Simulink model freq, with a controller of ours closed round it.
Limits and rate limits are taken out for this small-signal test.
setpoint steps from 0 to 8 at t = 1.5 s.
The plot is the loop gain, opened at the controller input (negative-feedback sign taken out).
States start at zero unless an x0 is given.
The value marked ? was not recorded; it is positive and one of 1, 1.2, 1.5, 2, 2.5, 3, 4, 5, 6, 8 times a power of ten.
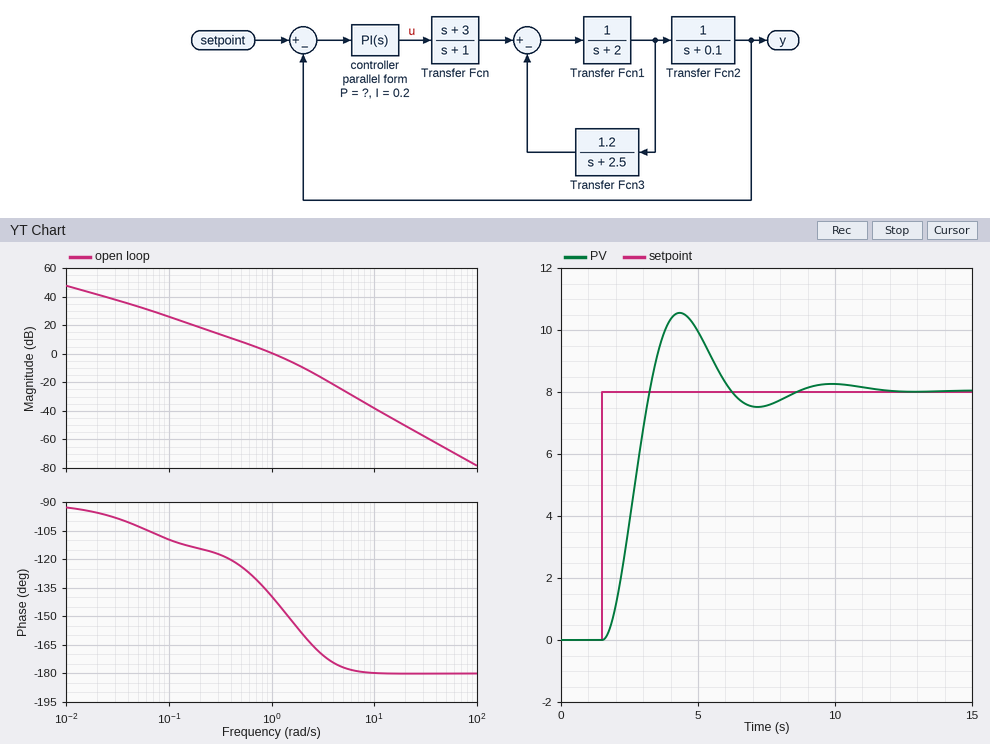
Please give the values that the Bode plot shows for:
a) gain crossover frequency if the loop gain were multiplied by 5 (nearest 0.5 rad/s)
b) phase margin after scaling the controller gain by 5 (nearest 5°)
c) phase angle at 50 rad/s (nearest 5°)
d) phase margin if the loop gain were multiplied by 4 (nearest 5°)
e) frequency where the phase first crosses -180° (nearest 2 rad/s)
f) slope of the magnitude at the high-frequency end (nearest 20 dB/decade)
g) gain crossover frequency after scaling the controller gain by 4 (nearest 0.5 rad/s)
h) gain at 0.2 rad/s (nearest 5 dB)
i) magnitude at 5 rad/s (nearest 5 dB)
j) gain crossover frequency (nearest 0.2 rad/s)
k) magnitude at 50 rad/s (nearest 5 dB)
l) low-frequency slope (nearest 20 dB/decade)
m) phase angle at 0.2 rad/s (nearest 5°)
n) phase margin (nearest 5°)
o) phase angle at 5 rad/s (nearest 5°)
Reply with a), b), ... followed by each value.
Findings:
a) 2.5 rad/s
b) 15°
c) -180°
d) 15°
e) 12 rad/s
f) -40 dB/decade
g) 2.5 rad/s
h) 20 dB
i) -25 dB
j) 1.0 rad/s
k) -65 dB
l) -20 dB/decade
m) -115°
n) 40°
o) -175°
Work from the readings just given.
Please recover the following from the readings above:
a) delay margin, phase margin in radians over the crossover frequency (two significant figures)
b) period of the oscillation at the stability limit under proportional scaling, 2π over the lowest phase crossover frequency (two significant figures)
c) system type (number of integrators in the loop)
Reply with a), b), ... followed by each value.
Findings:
a) 0.70 s
b) 0.52 s
c) 1
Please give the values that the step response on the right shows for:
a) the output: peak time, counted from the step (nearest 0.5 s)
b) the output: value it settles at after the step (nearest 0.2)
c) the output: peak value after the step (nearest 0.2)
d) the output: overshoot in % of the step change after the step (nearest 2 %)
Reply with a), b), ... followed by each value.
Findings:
a) 3.0 s
b) 8.0
c) 10.6
d) 32 %
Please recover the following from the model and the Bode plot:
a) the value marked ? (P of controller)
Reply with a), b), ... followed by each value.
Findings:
a) 1.2
